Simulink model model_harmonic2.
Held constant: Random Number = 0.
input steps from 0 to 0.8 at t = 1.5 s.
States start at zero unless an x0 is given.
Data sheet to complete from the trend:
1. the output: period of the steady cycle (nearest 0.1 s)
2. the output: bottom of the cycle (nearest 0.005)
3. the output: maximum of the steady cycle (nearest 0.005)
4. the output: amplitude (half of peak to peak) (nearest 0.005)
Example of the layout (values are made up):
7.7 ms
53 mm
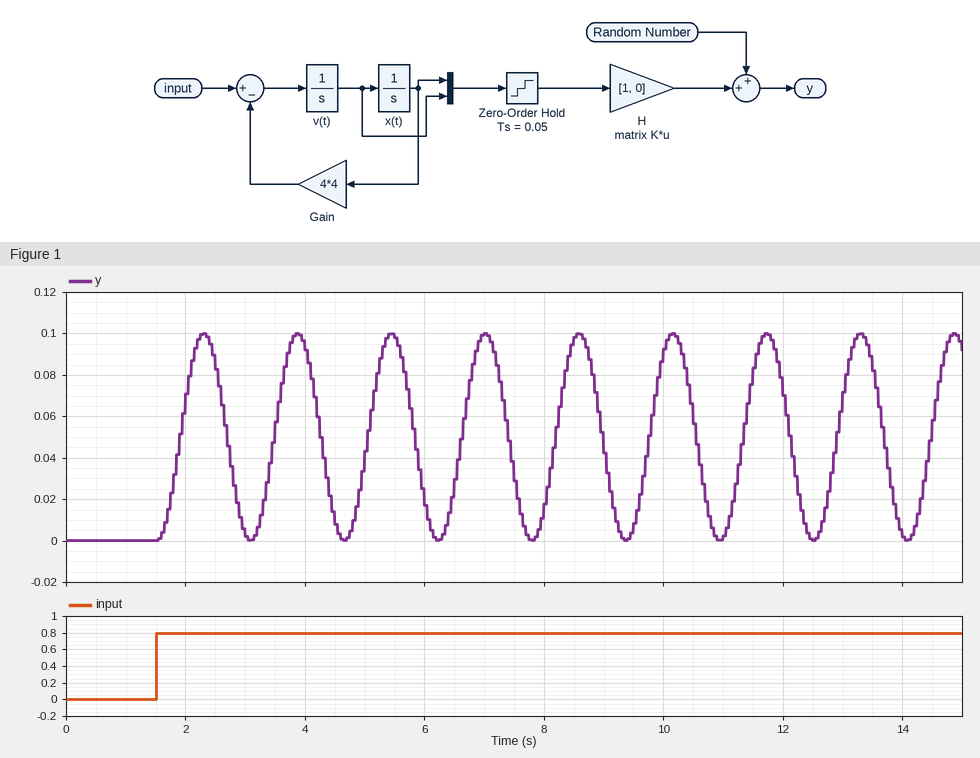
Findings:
1.6 s
0.000
0.100
0.050
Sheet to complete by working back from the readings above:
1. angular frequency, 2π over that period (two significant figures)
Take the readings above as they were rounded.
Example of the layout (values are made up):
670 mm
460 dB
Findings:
3.9 rad/s
